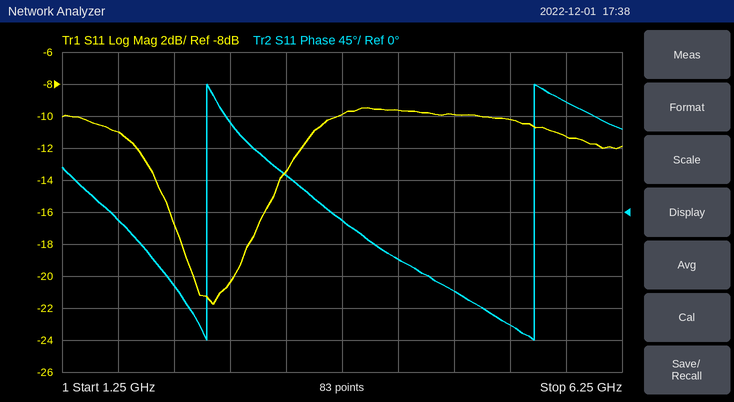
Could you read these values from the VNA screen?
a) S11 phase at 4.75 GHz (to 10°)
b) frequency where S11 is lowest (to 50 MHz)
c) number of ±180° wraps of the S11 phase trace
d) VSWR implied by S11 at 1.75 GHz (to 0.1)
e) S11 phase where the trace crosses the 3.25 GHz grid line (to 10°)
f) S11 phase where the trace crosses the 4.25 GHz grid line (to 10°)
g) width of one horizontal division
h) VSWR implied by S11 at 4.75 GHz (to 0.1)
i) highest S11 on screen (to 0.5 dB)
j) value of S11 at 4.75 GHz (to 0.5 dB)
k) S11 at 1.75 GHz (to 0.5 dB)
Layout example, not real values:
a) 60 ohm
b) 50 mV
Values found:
a) -110°
b) 2.60 GHz
c) 2
d) 1.8
e) 50°
f) -70°
g) 500 MHz
h) 1.9
i) -9.5 dB
j) -10.0 dB
k) -11.0 dB
